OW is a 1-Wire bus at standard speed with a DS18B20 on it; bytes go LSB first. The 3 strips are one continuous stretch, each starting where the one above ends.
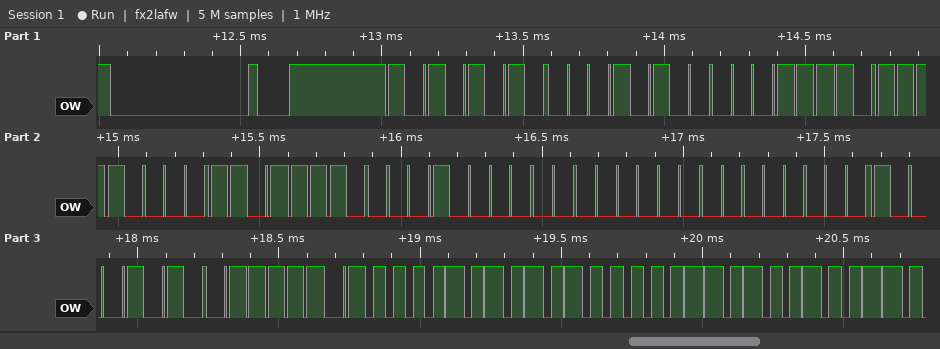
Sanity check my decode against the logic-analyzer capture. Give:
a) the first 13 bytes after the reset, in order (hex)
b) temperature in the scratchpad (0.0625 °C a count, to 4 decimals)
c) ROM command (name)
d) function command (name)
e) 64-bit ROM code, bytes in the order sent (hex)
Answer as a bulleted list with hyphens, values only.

- 55 28 78 0F 7B 08 00 00 51 BE 50 05 4B
- 85.0000 °C
- Match ROM
- Read Scratchpad
- 28 78 0F 7B 08 00 00 51
